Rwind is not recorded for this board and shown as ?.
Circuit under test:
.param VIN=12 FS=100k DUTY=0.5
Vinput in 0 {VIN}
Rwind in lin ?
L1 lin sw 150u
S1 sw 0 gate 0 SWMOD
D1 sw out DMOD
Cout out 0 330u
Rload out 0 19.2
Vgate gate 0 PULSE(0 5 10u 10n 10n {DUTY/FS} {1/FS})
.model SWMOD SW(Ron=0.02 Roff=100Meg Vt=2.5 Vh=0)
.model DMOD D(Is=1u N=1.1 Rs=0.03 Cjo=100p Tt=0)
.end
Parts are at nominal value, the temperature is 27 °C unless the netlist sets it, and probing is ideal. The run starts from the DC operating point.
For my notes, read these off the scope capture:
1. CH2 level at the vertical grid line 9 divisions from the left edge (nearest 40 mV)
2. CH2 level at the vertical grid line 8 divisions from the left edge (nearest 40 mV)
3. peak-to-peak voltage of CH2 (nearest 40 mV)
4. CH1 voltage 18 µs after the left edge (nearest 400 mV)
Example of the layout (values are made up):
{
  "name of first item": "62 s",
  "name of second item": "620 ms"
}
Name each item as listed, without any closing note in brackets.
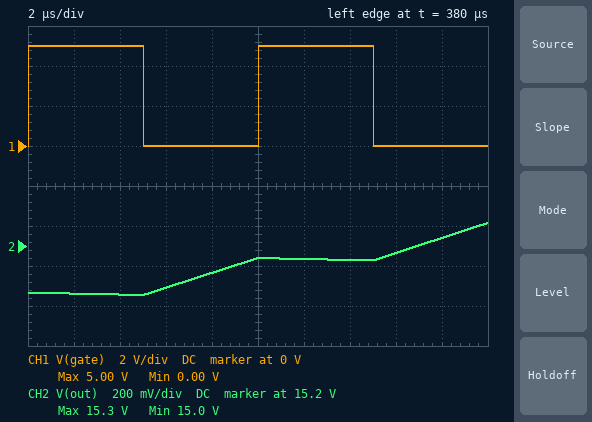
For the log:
{
  "CH2 level at the vertical grid line 9 divisions from the left edge": "15.24 V",
  "CH2 level at the vertical grid line 8 divisions from the left edge": "15.16 V",
  "peak-to-peak voltage of CH2": "360 mV",
  "CH1 voltage 18 µs after the left edge": "0 V"
}
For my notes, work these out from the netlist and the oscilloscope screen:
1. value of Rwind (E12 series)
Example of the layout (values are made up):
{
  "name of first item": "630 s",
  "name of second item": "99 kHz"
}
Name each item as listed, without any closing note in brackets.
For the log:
{
  "value of Rwind": "0.047 Ω"
}
